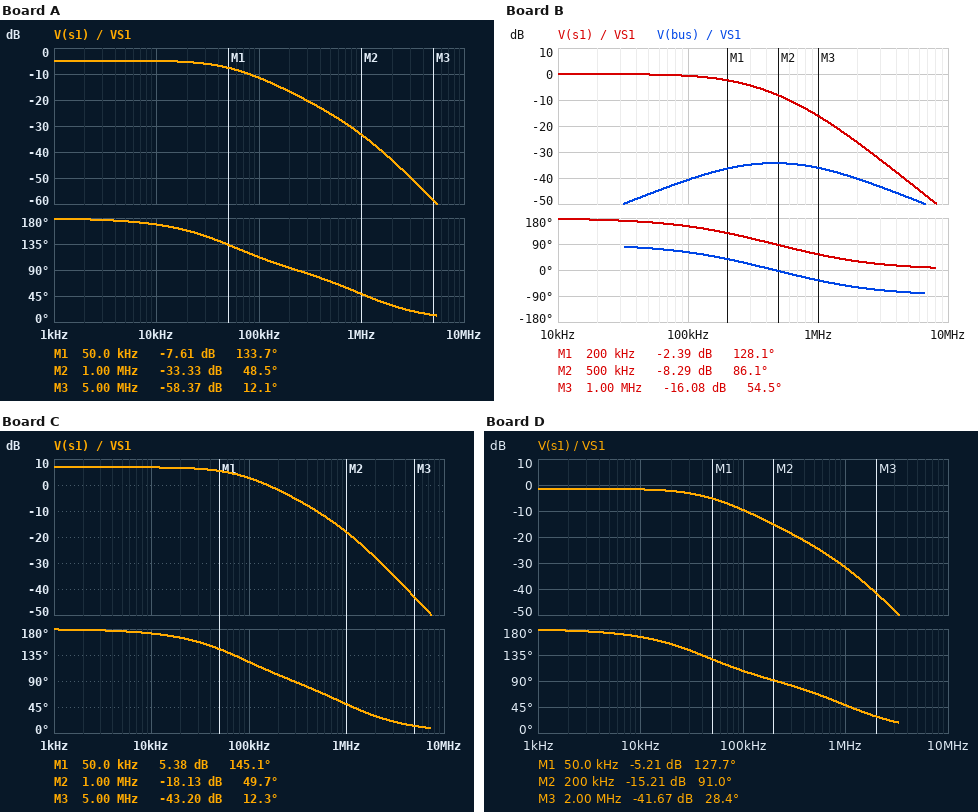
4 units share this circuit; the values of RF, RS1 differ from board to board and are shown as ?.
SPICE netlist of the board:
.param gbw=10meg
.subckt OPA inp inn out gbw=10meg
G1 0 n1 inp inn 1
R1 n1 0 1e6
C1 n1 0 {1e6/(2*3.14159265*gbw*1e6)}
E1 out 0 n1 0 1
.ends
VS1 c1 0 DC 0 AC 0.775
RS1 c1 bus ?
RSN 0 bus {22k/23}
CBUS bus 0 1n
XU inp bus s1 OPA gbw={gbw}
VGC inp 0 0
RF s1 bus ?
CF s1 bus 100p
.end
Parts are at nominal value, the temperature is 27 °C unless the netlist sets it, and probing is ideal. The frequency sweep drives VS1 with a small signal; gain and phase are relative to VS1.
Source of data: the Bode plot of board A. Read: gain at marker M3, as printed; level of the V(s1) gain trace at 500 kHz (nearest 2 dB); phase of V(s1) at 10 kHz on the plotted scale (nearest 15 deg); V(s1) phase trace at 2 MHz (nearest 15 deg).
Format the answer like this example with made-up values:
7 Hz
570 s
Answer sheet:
-58.37 dB
-26 dB
165 deg
30 deg
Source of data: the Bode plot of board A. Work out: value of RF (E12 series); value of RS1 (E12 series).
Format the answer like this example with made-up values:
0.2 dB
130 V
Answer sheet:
27 kΩ
47 kΩ
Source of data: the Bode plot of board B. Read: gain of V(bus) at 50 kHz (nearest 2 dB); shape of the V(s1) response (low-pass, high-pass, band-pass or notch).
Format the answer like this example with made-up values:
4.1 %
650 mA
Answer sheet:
-46 dB
low-pass
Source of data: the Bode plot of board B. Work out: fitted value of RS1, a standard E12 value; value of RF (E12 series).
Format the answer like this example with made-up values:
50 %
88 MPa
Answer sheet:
6.8 kΩ
6.8 kΩ
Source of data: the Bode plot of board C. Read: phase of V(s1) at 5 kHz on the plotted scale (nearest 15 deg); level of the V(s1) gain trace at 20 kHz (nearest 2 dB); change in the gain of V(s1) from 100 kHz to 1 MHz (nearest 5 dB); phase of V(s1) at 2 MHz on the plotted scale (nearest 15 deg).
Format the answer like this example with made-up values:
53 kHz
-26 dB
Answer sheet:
180 deg
6 dB
-20 dB
30 deg
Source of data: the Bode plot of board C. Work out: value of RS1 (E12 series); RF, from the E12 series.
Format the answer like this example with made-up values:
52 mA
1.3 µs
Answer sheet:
8.2 kΩ
18 kΩ
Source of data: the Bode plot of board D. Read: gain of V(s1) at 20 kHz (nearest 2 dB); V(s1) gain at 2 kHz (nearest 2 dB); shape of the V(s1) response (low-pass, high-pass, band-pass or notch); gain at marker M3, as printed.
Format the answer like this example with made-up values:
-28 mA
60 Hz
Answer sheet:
-2 dB
-2 dB
low-pass
-41.67 dB
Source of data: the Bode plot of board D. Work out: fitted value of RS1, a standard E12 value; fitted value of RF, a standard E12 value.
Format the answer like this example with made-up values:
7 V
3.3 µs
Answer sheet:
39 kΩ
33 kΩ
